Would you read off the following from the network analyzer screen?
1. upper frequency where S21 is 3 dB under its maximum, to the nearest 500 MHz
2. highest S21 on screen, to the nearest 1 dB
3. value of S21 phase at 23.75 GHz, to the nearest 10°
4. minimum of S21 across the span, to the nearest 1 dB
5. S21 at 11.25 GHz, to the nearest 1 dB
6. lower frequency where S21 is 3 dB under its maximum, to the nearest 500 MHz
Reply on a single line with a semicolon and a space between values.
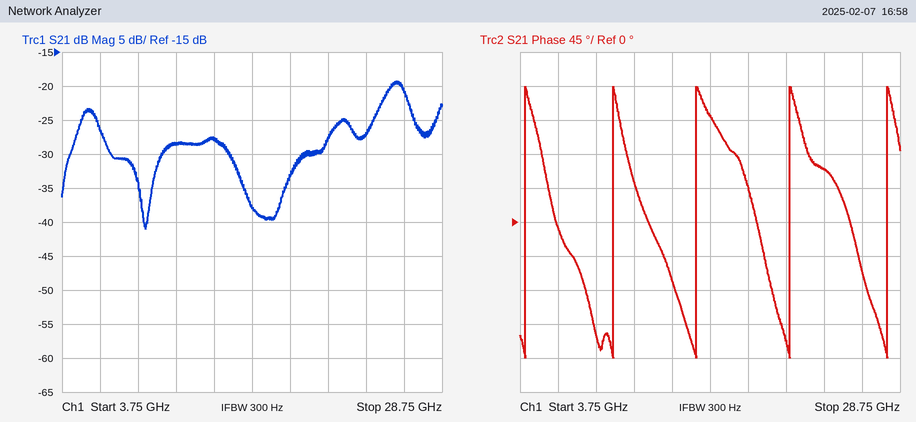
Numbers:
26.5 GHz; -19 dB; 70°; -41 dB; -28 dB; 25.0 GHz
